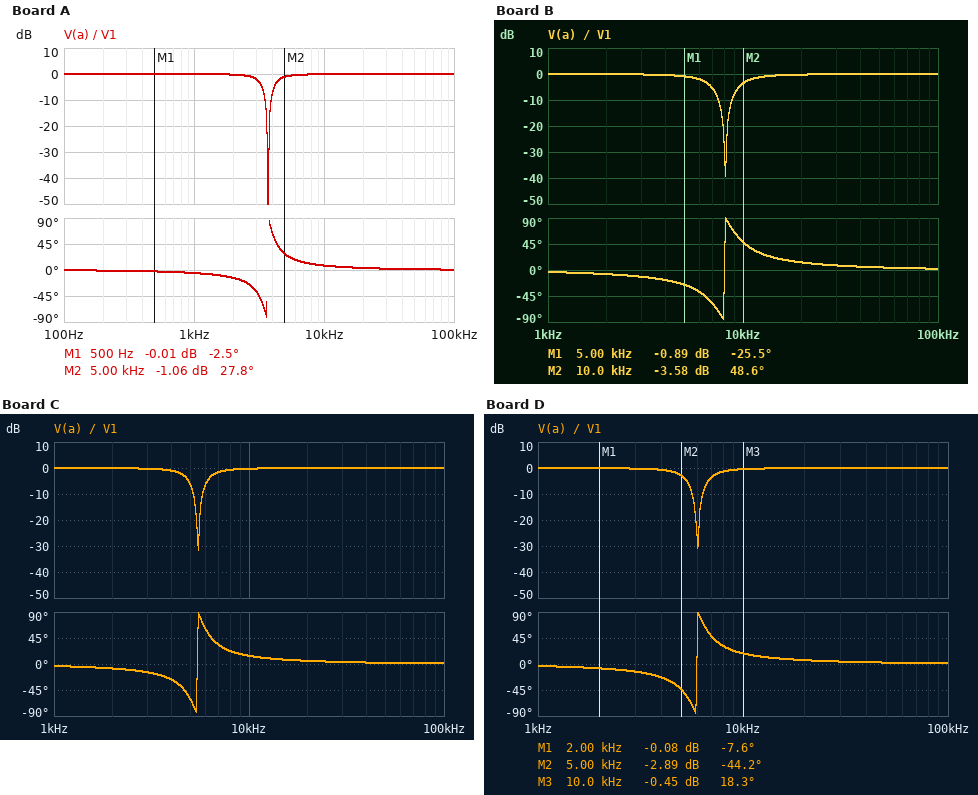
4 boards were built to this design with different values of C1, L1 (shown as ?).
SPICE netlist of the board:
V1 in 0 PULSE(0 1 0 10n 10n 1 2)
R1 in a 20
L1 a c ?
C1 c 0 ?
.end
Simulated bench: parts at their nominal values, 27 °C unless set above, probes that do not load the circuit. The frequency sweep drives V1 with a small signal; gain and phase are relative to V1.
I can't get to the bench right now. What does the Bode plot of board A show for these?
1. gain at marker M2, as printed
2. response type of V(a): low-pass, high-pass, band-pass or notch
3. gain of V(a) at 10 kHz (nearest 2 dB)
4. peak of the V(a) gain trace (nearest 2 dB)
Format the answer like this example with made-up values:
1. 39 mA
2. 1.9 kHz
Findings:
1. -1.06 dB
2. notch
3. 0 dB
4. 0 dB
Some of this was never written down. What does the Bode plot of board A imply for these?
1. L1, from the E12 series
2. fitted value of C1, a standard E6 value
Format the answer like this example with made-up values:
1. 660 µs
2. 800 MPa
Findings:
1. 2.7 mH
2. 680 nF
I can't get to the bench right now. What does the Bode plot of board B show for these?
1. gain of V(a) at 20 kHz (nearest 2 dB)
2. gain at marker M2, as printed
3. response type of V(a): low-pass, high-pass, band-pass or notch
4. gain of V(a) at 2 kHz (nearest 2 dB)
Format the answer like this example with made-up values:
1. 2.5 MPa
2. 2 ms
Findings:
1. 0 dB
2. -3.58 dB
3. notch
4. 0 dB
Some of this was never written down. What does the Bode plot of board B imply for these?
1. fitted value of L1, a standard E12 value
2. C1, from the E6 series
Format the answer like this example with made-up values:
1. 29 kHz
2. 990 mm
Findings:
1. 820 µH
2. 470 nF
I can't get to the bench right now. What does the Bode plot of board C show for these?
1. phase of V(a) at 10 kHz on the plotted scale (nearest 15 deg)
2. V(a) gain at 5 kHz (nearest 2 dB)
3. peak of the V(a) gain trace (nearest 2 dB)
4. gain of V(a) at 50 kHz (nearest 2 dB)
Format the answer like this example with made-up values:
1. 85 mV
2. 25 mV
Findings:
1. 15 deg
2. -6 dB
3. 0 dB
4. 0 dB
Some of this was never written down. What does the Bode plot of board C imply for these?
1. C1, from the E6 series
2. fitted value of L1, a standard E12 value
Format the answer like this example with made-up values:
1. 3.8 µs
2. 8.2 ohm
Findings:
1. 470 nF
2. 1.8 mH
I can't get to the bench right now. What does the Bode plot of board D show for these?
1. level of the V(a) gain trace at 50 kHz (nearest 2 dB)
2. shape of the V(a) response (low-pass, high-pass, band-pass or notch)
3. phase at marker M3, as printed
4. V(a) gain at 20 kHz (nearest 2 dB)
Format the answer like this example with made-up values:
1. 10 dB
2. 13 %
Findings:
1. 0 dB
2. notch
3. 18.3 deg
4. 0 dB
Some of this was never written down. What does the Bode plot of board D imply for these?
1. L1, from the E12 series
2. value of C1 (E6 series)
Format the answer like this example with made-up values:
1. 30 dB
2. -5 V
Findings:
1. 1.5 mH
2. 470 nF
